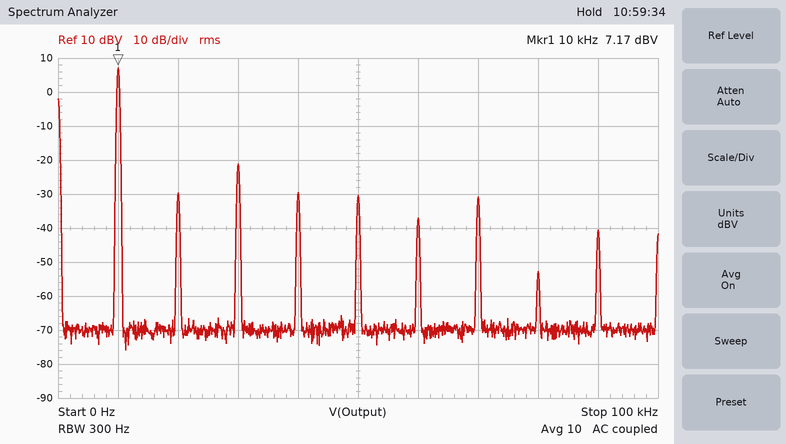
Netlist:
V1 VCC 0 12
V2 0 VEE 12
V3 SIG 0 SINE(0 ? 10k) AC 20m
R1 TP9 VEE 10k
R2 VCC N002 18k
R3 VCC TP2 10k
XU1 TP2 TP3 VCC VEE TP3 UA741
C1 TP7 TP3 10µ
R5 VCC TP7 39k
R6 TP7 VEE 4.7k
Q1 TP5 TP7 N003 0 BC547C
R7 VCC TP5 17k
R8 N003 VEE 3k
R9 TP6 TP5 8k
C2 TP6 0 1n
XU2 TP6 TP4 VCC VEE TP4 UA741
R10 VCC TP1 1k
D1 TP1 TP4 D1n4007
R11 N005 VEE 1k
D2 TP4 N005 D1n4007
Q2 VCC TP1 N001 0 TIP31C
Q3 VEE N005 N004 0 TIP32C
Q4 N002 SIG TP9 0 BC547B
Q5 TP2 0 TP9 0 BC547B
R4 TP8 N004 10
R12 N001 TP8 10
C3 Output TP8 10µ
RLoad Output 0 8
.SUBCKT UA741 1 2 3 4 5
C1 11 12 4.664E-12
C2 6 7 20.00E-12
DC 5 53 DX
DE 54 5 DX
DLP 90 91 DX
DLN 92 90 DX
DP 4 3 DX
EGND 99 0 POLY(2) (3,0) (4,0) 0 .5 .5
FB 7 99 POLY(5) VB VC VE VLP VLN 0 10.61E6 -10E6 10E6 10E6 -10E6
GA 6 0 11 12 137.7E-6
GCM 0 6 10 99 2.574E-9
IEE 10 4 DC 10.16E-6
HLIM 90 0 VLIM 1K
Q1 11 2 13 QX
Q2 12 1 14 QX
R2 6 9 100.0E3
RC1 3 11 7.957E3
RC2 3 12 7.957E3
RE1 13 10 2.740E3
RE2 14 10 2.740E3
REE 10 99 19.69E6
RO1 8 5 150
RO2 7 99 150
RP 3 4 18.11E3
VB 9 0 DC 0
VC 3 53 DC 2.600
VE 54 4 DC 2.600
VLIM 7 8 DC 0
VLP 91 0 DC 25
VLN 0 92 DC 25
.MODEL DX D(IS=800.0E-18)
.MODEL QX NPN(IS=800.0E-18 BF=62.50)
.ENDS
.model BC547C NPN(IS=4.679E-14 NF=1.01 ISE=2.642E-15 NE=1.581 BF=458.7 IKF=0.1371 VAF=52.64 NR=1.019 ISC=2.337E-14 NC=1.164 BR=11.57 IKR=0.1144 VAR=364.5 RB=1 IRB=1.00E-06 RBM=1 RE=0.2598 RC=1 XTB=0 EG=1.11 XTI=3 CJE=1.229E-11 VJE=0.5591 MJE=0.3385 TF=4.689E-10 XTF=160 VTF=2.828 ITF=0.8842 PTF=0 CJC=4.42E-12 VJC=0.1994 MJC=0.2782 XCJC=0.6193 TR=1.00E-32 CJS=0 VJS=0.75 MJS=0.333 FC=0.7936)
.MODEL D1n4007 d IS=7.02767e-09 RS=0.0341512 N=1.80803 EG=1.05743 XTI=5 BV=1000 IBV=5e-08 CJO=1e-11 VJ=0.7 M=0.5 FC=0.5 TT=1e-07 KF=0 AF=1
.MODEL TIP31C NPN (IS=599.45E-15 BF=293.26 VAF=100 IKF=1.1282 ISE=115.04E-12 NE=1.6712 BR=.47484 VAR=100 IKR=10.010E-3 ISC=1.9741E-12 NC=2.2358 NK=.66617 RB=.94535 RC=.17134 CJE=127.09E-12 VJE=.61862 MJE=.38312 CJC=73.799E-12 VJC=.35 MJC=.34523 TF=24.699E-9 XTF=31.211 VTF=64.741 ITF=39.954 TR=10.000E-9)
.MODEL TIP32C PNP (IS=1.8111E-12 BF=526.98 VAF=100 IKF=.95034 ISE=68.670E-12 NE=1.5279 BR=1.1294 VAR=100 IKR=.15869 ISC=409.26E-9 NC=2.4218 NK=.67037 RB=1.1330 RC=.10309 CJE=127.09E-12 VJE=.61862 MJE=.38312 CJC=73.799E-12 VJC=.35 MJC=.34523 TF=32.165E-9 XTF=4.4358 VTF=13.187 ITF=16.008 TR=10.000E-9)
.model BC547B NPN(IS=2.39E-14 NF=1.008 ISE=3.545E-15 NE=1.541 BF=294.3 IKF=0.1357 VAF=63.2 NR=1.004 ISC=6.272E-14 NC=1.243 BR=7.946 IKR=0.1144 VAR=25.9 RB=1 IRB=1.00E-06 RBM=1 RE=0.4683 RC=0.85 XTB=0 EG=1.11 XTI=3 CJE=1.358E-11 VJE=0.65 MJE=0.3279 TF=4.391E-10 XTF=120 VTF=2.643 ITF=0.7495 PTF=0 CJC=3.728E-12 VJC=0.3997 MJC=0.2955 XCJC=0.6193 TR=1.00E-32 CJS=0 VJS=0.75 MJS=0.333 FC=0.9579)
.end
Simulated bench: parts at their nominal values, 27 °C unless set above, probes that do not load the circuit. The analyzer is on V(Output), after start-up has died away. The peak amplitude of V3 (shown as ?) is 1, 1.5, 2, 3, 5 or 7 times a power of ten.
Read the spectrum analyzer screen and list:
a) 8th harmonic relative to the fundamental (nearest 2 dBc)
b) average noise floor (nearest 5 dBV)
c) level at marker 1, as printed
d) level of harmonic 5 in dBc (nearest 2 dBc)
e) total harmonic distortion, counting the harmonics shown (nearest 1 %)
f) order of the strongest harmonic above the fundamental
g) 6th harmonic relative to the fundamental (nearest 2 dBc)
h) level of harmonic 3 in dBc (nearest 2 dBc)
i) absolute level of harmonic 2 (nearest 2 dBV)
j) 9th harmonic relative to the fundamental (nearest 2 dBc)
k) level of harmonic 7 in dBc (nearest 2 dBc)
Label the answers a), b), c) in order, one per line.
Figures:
a) -60 dBc
b) -70 dBV
c) 7.17 dBV
d) -38 dBc
e) 5 %
f) 3
g) -44 dBc
h) -28 dBc
i) -30 dBV
j) -48 dBc
k) -38 dBc
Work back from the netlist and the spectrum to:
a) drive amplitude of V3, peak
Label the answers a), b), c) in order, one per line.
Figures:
a) 50 mV
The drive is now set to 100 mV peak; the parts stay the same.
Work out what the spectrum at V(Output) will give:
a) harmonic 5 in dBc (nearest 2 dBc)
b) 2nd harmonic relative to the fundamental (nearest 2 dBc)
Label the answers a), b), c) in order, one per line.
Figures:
a) -32 dBc
b) -34 dBc
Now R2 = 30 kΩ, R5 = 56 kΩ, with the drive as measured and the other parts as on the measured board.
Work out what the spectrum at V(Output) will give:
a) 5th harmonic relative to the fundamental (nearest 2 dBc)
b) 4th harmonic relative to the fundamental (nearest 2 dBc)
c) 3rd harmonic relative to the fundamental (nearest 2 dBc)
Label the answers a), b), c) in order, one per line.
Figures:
a) -40 dBc
b) -38 dBc
c) -42 dBc
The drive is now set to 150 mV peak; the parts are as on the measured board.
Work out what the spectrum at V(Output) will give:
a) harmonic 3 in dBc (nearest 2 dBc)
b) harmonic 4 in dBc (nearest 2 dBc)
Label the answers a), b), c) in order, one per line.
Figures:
a) -32 dBc
b) -34 dBc
